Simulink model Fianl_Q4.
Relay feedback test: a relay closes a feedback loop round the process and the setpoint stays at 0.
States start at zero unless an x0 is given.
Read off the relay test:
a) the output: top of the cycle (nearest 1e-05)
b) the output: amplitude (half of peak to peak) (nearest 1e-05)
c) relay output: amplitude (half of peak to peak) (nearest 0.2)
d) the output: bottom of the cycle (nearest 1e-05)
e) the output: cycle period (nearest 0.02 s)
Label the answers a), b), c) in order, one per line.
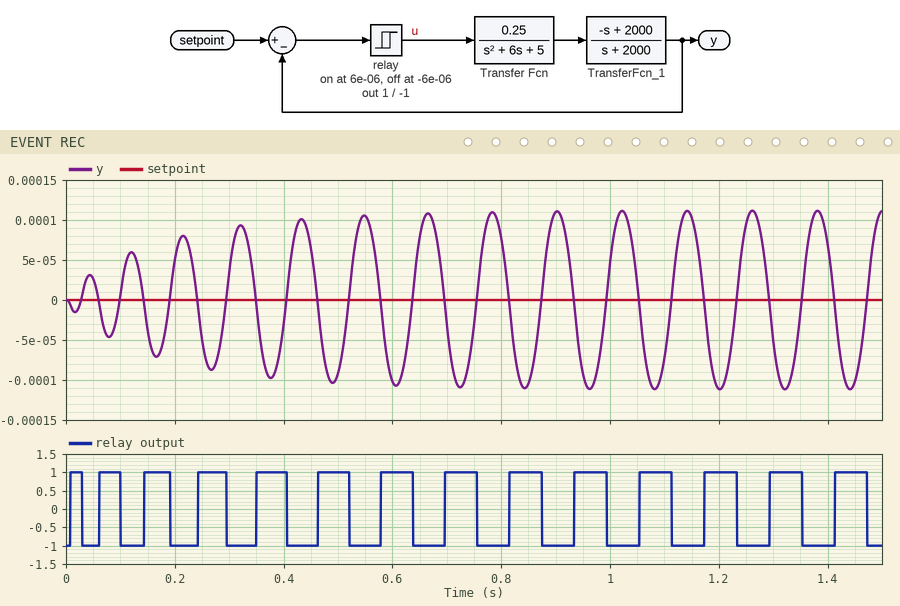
a) 0.00011
b) 0.00011
c) 1.0
d) -0.00011
e) 0.12 s
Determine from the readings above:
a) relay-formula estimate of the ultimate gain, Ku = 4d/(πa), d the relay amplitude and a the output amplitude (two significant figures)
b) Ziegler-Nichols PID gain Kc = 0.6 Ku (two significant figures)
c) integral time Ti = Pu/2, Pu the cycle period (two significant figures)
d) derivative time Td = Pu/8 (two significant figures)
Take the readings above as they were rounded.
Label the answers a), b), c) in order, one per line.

a) 12000
b) 7200
c) 0.060 s
d) 0.015 s
